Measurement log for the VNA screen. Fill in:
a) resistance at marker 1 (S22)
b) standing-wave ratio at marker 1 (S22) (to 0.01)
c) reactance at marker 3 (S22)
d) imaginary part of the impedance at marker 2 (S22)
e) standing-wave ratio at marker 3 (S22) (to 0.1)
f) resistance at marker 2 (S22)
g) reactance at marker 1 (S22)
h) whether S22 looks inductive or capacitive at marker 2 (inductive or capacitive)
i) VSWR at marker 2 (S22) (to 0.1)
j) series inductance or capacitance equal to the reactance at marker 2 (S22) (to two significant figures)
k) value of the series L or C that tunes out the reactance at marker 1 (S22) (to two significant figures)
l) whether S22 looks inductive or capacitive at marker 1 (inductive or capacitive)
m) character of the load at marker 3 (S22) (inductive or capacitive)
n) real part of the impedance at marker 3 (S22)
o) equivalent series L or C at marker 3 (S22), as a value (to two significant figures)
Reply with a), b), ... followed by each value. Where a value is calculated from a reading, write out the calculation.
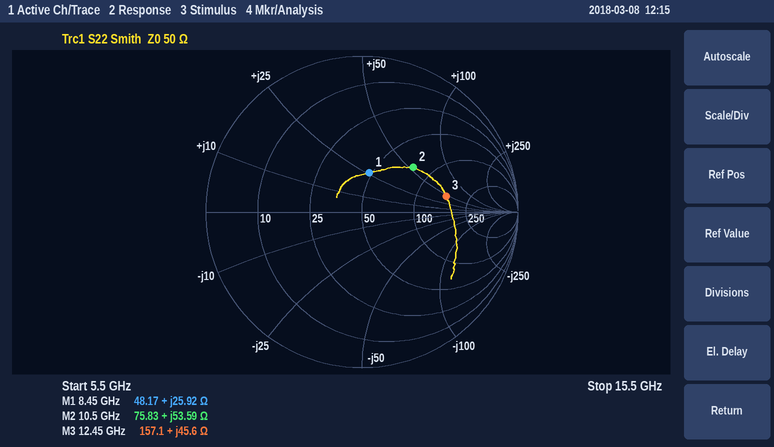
a) 48.17 Ω
b) 1.69
c) +45.6 Ω
d) +53.59 Ω
e) 3.4
f) 75.83 Ω
g) +25.92 Ω
h) inductive
i) 2.5
j) L = 53.59 Ω/(2π × 10.5 GHz) ≈ 812 pH, so 810 pH to two significant figures
k) C = 1/(2π × 8.45 GHz × 25.92 Ω) ≈ 727 fF, so 730 fF to two significant figures
l) inductive
m) inductive
n) 157.1 Ω
o) L = 45.6 Ω/(2π × 12.45 GHz) ≈ 583 pH, so 580 pH to two significant figures
